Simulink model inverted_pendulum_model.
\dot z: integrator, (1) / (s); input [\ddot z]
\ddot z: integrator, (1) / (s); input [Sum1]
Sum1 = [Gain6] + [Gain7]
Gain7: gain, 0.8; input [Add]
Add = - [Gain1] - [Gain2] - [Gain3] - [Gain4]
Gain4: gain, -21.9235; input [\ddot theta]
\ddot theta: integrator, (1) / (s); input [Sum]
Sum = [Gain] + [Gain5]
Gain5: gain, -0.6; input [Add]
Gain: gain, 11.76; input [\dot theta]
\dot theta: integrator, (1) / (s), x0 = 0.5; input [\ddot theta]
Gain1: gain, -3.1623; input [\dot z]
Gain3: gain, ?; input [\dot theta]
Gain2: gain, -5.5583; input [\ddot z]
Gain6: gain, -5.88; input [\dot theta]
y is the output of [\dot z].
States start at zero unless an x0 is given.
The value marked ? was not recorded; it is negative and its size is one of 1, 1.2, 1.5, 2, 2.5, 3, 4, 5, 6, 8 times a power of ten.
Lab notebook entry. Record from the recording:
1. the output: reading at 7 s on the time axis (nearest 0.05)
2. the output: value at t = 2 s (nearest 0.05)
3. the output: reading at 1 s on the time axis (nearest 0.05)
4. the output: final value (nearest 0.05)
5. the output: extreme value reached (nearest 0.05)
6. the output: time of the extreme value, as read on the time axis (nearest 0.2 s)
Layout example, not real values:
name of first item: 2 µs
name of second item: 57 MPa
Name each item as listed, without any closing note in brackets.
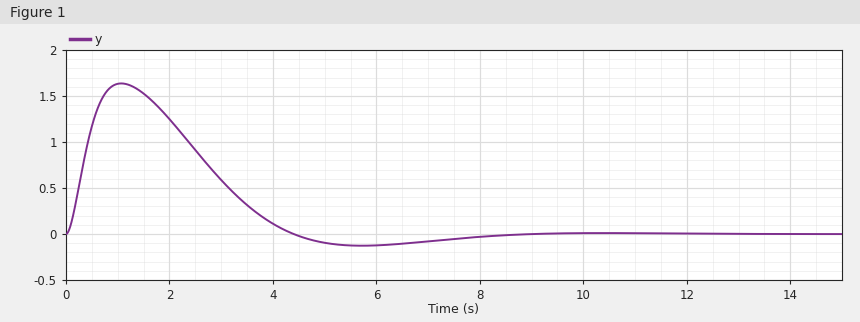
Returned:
the output: reading at 7 s on the time axis: -0.10
the output: value at t = 2 s: 1.25
the output: reading at 1 s on the time axis: 1.65
the output: final value: 0.00
the output: extreme value reached: 1.65
the output: time of the extreme value, as read on the time axis: 1.0 s
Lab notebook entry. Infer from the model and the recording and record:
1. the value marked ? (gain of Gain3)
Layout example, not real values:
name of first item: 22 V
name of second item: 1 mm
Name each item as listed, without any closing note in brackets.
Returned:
the value marked ?: -80
